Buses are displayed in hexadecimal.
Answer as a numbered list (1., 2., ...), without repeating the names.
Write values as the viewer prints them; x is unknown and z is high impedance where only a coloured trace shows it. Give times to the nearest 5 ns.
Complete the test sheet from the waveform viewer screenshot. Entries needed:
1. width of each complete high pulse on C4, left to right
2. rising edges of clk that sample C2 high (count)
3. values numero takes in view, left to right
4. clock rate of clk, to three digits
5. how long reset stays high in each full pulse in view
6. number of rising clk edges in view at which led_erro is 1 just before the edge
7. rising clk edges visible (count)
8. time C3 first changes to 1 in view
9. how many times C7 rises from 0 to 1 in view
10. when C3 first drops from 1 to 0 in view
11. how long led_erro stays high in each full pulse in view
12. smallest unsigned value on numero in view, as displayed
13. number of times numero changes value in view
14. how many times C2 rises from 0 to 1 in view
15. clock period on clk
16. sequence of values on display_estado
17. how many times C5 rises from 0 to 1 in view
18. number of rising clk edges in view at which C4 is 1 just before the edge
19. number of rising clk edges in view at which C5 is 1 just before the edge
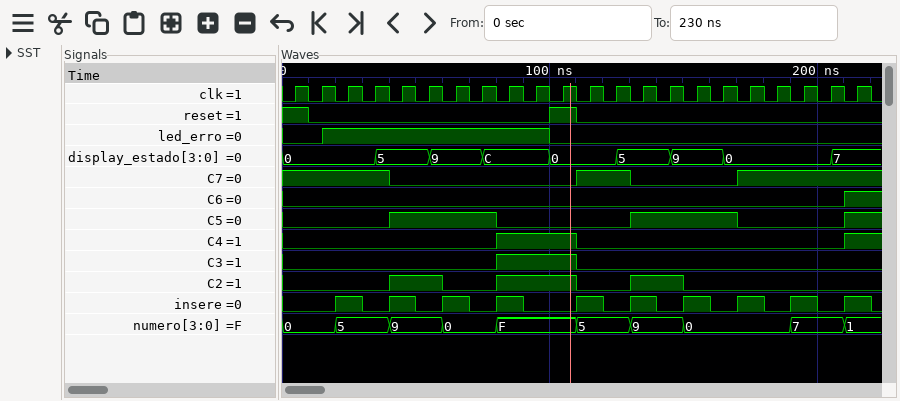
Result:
1. 30 ns
2. 7
3. 0, 5, 9, 0, F, 5, 9, 0, 7, 1
4. 100 MHz
5. 10 ns
6. 8
7. 22
8. 80 ns
9. 2
10. 110 ns
11. 85 ns
12. 0
13. 9
14. 3
15. 10 ns
16. 0, 5, 9, C, 0, 5, 9, 0, 7
17. 3
18. 4
19. 9
